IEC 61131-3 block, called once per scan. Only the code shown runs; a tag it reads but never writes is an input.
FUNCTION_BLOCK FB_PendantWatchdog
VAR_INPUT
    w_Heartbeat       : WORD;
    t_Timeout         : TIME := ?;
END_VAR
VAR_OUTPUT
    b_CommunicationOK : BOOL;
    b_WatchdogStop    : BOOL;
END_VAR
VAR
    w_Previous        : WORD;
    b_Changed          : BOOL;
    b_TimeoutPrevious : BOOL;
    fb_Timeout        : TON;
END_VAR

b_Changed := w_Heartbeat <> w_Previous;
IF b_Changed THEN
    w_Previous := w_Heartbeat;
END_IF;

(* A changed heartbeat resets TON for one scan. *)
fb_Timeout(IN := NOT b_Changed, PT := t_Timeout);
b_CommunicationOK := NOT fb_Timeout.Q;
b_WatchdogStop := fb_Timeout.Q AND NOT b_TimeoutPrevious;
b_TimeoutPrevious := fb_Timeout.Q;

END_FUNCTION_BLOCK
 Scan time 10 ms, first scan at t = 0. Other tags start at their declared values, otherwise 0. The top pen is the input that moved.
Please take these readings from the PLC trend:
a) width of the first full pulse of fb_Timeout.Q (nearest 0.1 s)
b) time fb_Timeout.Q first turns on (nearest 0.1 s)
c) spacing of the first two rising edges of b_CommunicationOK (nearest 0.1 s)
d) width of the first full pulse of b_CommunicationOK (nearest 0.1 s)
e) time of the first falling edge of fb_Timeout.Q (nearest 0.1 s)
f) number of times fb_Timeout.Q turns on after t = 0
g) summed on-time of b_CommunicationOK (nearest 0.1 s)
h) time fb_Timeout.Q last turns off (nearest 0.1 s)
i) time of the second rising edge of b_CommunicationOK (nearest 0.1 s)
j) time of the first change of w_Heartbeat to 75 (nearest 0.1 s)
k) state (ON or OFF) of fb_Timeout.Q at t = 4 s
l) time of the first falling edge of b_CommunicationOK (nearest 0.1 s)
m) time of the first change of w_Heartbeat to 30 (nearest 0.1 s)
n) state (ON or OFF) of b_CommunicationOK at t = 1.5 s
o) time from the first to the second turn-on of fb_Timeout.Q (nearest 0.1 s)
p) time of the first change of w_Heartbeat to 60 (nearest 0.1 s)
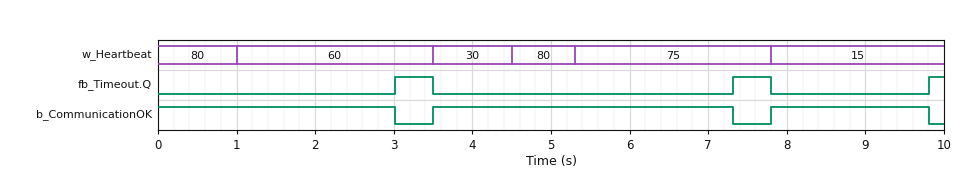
0.5 s
3.0 s
4.3 s
3.8 s
3.5 s
3
8.8 s
7.8 s
7.8 s
5.3 s
OFF
3.0 s
3.5 s
ON
4.3 s
1.0 s
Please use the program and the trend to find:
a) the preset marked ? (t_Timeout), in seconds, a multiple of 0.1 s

2.0 s
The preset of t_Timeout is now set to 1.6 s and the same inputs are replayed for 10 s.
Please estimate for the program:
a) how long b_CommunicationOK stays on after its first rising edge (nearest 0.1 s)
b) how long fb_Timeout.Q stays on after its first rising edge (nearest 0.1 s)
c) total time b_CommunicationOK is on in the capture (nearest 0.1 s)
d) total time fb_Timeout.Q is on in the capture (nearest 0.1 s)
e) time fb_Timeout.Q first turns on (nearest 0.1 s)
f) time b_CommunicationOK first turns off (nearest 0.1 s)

3.4 s
0.9 s
7.6 s
2.4 s
2.6 s
2.6 s
